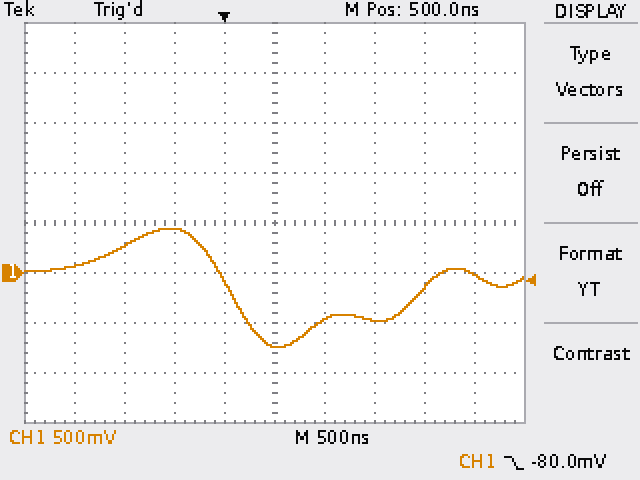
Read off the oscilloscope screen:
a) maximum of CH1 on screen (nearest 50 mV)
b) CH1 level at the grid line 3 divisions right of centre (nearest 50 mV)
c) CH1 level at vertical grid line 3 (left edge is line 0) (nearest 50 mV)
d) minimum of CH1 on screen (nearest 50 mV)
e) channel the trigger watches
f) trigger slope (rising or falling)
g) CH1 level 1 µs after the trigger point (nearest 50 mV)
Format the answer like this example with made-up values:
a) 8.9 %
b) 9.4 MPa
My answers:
a) 450 mV
b) -150 mV
c) 450 mV
d) -750 mV
e) CH1
f) falling
g) -450 mV
